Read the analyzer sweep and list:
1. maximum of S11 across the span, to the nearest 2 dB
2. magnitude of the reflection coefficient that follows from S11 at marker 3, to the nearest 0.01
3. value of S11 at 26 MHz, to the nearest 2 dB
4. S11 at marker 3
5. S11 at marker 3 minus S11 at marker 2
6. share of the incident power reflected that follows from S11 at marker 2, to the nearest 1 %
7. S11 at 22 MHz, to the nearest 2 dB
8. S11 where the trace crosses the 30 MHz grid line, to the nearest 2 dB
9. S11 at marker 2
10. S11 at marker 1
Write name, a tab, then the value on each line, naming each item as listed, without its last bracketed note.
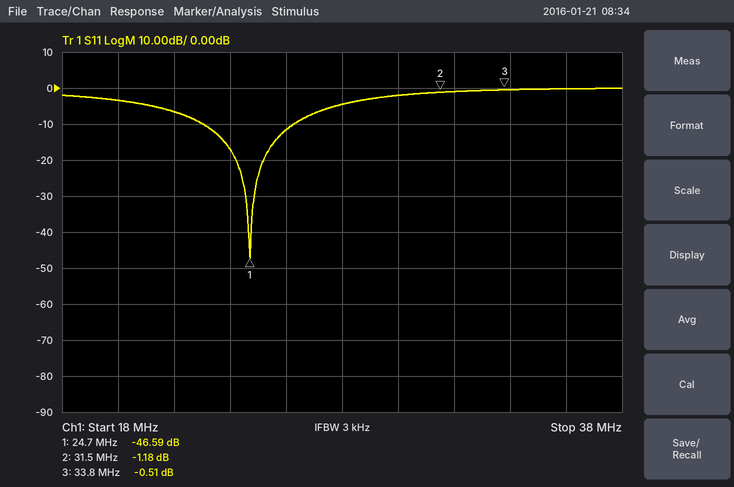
maximum of S11 across the span, to the nearest 2 dB	0 dB
magnitude of the reflection coefficient that follows from S11 at marker 3, to the nearest 0.01	0.94
value of S11 at 26 MHz, to the nearest 2 dB	-12 dB
S11 at marker 3	-0.51 dB
S11 at marker 3 minus S11 at marker 2	0.67 dB
share of the incident power reflected that follows from S11 at marker 2, to the nearest 1 %	76 %
S11 at 22 MHz, to the nearest 2 dB	-6 dB
S11 where the trace crosses the 30 MHz grid line, to the nearest 2 dB	-2 dB
S11 at marker 2	-1.18 dB
S11 at marker 1	-46.59 dB
